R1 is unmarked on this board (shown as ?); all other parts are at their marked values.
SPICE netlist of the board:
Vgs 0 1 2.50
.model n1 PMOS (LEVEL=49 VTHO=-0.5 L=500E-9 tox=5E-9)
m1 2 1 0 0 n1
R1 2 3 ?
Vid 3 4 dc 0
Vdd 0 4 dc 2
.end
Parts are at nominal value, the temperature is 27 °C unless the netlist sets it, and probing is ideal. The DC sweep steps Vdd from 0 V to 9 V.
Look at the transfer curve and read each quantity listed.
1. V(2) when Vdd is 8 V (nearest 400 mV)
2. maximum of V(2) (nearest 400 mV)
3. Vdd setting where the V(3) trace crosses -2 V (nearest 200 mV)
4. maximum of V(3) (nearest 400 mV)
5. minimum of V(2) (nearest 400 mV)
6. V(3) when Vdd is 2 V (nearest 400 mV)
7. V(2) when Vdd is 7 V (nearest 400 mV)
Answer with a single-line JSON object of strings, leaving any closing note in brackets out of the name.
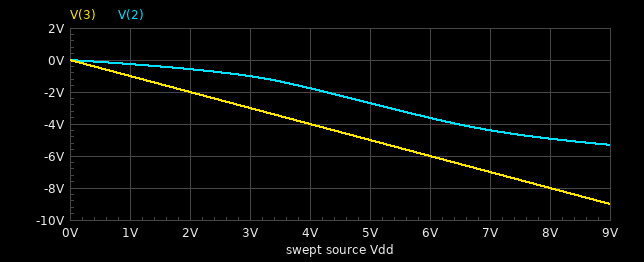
{"V(2) when Vdd is 8 V": "-4.8 V", "maximum of V(2)": "0 V", "Vdd setting where the V(3) trace crosses -2 V": "2.0 V", "maximum of V(3)": "0 V", "minimum of V(2)": "-5.2 V", "V(3) when Vdd is 2 V": "-2.0 V", "V(2) when Vdd is 7 V": "-4.4 V"}
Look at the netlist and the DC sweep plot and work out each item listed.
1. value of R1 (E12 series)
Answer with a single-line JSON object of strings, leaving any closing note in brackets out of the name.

{"value of R1": "2.7 kΩ"}
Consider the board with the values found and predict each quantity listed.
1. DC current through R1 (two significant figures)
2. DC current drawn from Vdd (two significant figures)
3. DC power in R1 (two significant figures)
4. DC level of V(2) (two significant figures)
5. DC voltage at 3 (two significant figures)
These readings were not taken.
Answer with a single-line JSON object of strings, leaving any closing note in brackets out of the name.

{"DC current through R1": "530 µA", "DC current drawn from Vdd": "530 µA", "DC power in R1": "760 µW", "DC level of V(2)": "-570 mV", "DC voltage at 3": "-2.0 V"}
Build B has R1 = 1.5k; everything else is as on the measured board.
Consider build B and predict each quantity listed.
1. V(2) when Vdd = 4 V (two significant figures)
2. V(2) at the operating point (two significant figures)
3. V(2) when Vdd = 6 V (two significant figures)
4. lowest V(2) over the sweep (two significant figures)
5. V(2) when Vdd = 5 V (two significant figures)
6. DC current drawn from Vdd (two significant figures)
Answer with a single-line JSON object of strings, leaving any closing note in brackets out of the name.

{"V(2) when Vdd = 4 V": "-2.7 V", "V(2) at the operating point": "-930 mV", "V(2) when Vdd = 6 V": "-4.5 V", "lowest V(2) over the sweep": "-6.0 V", "V(2) when Vdd = 5 V": "-3.7 V", "DC current drawn from Vdd": "710 µA"}
